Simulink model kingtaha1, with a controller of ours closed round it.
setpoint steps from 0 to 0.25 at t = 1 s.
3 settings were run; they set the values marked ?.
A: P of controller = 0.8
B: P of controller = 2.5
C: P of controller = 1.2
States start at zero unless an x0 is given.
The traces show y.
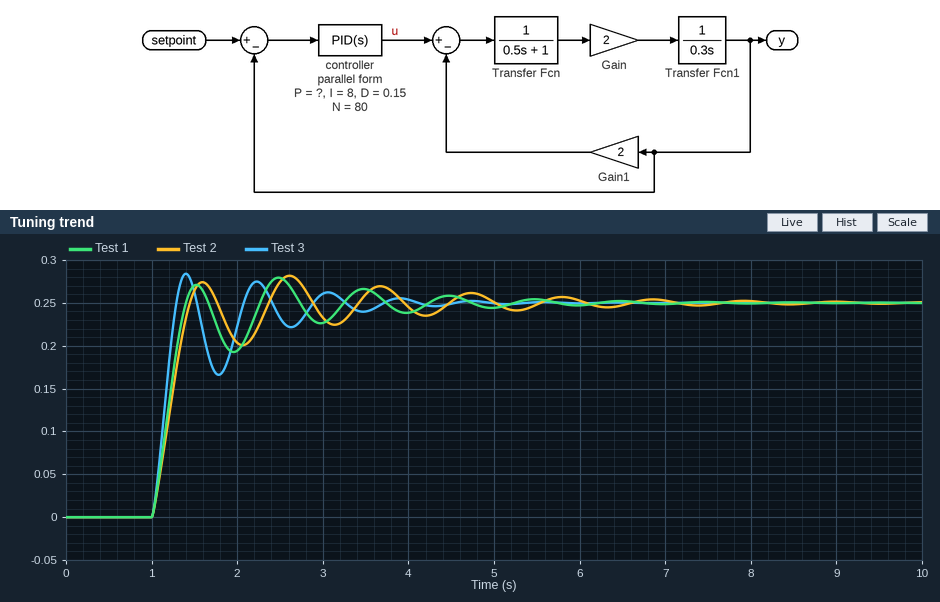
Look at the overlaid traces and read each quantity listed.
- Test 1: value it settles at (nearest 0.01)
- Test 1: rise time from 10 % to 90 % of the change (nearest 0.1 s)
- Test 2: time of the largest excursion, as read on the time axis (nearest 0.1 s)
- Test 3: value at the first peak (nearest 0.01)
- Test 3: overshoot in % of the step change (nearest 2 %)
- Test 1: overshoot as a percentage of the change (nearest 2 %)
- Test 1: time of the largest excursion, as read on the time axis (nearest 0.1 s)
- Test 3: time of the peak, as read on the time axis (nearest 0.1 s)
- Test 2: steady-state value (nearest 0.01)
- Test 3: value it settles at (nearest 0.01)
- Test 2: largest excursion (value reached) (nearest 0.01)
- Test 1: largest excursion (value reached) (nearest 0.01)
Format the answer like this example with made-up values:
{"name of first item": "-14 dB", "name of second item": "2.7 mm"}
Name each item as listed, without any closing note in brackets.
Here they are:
{"Test 1: value it settles at": "0.25", "Test 1: rise time from 10 % to 90 % of the change": "0.3 s", "Test 2: time of the largest excursion, as read on the time axis": "2.6 s", "Test 3: value at the first peak": "0.28", "Test 3: overshoot in % of the step change": "14 %", "Test 1: overshoot as a percentage of the change": "12 %", "Test 1: time of the largest excursion, as read on the time axis": "2.5 s", "Test 3: time of the peak, as read on the time axis": "1.4 s", "Test 2: steady-state value": "0.25", "Test 3: value it settles at": "0.25", "Test 2: largest excursion (value reached)": "0.28", "Test 1: largest excursion (value reached)": "0.28"}
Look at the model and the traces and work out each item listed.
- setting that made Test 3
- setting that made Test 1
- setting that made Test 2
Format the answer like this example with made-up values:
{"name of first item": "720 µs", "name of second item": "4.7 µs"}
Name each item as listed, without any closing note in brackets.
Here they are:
{"setting that made Test 3": "B", "setting that made Test 1": "C", "setting that made Test 2": "A"}
